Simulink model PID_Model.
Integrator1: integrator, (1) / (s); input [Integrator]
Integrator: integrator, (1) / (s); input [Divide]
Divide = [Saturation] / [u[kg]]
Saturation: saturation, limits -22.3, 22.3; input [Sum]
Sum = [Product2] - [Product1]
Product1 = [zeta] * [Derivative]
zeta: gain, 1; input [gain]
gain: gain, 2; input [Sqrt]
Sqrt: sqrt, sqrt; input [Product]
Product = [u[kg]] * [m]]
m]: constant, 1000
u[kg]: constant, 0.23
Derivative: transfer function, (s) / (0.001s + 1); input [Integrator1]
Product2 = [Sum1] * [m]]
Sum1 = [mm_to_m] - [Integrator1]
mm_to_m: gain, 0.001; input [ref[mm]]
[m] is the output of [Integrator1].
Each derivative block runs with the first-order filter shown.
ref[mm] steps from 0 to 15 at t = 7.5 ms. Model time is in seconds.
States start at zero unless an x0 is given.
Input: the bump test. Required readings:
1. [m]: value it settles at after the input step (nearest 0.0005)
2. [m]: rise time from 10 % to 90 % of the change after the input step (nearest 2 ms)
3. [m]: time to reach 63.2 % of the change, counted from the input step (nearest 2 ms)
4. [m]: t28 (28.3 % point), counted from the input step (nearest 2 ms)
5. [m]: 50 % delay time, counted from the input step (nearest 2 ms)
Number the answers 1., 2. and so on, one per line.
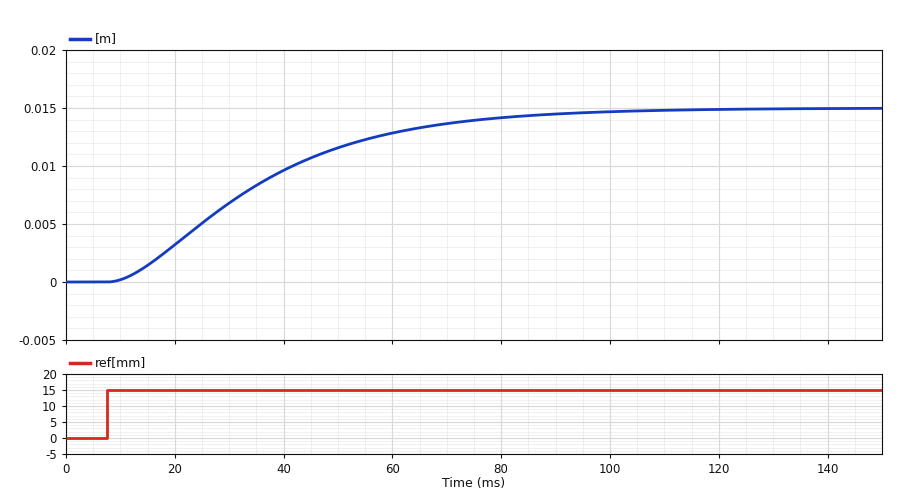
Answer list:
1. 0.0150
2. 52 ms
3. 32 ms
4. 16 ms
5. 24 ms
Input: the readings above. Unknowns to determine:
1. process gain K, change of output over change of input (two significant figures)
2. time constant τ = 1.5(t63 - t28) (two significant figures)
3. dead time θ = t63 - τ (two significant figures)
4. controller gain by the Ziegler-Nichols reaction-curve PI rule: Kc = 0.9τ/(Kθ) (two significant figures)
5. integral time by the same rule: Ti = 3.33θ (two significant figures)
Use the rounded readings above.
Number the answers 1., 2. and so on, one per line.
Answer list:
1. 0.0010
2. 24 ms
3. 8.0 ms
4. 2700
5. 27 ms
